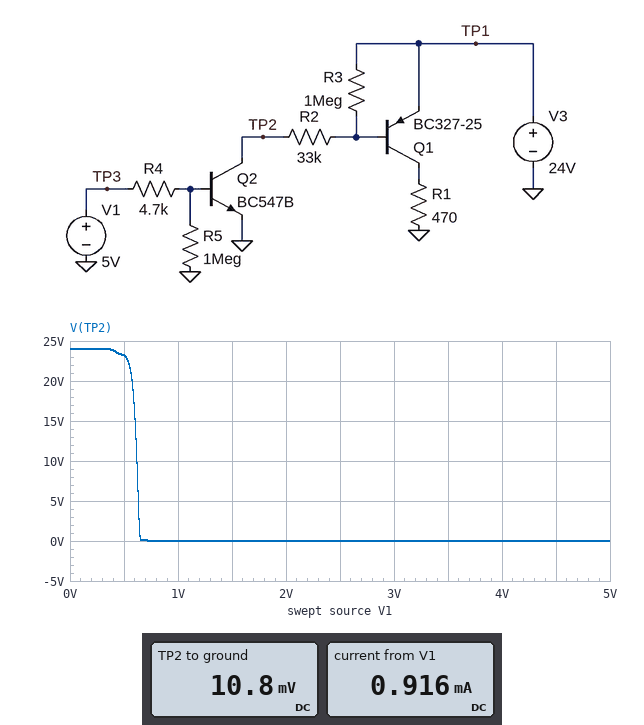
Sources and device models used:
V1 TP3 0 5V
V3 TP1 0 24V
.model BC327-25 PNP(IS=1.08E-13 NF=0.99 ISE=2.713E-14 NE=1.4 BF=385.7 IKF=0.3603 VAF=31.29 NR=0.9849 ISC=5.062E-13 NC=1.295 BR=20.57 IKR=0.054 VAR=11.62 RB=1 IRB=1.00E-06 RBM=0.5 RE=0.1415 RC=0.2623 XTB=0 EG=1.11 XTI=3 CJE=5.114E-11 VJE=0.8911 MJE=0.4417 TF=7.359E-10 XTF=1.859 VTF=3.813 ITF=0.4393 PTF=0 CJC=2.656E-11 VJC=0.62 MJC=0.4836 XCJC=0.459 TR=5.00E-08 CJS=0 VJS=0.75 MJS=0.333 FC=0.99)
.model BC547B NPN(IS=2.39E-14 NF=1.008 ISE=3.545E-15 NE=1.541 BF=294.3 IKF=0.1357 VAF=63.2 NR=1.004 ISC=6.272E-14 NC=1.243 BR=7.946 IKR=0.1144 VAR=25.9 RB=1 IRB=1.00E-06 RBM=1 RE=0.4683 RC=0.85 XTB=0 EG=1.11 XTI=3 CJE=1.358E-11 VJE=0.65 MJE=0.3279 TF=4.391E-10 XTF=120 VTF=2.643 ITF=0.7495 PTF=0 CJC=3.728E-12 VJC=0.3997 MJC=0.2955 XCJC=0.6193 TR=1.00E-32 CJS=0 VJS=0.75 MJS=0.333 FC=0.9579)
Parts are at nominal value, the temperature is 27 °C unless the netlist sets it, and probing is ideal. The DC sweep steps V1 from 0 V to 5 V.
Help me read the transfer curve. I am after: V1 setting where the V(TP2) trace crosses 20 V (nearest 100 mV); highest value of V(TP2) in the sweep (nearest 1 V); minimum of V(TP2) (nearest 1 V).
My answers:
600 mV
24 V
0 V
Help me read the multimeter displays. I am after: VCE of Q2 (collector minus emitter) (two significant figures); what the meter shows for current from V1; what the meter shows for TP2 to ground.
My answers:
11 mV
0.916 mA
10.8 mV
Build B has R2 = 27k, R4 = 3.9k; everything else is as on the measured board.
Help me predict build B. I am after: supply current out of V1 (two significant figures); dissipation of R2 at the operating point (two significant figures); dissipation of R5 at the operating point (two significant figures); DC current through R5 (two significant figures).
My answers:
1.1 mA
20 mW
490 nW
700 nA
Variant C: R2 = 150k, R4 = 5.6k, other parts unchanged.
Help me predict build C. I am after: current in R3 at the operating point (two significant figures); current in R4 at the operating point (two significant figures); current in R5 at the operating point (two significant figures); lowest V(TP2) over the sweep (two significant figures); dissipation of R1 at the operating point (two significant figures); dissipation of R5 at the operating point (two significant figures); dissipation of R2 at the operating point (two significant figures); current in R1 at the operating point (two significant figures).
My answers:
700 nA
770 µA
690 nA
7.9 mV
1.1 W
470 nW
3.6 mW
48 mA
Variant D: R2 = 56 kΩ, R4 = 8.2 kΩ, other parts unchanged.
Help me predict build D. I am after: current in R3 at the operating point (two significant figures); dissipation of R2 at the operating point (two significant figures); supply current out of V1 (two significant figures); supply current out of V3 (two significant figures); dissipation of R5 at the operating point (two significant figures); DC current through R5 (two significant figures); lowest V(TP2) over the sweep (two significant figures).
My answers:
700 nA
9.7 mW
530 µA
51 mA
460 nW
680 nA
10 mV
